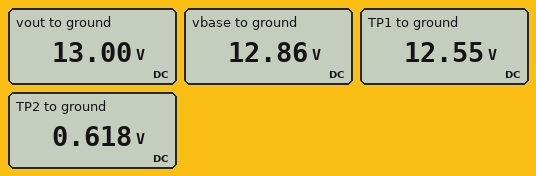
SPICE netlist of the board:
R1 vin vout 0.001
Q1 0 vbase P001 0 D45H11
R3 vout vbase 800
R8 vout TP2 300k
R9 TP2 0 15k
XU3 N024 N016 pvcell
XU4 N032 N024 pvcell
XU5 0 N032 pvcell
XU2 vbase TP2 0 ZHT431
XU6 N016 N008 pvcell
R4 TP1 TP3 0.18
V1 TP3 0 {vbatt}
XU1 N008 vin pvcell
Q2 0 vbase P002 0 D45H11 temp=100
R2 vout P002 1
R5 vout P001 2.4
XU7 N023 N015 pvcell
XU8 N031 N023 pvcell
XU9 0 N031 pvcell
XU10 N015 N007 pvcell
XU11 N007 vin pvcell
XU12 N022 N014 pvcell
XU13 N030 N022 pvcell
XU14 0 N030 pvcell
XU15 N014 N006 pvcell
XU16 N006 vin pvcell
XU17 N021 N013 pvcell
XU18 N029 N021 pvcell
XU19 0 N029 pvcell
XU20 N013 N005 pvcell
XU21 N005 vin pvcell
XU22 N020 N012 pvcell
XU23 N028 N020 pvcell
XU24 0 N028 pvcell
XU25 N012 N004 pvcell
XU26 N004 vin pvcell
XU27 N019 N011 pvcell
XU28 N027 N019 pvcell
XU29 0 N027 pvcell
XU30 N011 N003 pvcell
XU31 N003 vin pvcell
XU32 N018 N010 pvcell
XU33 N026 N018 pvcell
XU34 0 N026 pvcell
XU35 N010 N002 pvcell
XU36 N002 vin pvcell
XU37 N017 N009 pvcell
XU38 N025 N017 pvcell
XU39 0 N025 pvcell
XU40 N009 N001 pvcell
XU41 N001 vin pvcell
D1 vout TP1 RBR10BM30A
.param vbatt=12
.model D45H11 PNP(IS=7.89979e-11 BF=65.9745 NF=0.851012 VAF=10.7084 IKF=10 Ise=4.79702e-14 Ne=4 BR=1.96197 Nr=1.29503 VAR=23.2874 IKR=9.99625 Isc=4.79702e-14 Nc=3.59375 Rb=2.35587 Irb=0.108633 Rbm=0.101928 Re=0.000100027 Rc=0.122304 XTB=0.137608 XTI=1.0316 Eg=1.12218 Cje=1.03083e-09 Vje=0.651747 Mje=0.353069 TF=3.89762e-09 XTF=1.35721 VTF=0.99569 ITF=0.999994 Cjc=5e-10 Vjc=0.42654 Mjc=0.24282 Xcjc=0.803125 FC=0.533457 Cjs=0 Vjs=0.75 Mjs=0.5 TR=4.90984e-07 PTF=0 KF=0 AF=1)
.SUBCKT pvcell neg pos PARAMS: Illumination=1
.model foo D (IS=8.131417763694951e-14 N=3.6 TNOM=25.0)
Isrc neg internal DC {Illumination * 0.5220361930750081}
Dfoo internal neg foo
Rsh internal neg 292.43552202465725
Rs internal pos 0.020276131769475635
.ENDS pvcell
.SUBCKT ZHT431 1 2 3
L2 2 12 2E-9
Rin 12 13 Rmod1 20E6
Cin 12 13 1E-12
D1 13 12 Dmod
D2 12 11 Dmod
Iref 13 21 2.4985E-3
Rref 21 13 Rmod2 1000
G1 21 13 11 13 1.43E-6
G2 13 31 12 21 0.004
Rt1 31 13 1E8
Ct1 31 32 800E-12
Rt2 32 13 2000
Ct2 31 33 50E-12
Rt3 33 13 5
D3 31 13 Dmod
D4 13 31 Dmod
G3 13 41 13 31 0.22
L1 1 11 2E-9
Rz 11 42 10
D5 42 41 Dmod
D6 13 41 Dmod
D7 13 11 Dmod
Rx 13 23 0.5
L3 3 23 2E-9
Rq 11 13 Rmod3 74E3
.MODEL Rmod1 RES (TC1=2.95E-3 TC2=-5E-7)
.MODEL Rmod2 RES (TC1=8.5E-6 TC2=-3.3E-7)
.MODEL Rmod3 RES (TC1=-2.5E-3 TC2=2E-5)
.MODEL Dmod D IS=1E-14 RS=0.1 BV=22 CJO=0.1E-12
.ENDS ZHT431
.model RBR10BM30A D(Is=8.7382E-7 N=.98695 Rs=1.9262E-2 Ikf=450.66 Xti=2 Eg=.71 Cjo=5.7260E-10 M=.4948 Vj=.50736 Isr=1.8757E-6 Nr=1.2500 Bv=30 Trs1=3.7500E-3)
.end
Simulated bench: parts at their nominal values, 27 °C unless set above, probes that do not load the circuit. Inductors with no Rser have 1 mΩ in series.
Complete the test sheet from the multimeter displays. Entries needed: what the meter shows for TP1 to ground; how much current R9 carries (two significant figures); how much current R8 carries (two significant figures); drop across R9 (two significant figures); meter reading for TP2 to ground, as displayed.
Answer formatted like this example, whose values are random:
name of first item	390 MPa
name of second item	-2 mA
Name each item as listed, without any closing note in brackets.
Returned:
what the meter shows for TP1 to ground	12.55 V
how much current R9 carries	41 µA
how much current R8 carries	41 µA
drop across R9	620 mV
meter reading for TP2 to ground, as displayed	0.618 V
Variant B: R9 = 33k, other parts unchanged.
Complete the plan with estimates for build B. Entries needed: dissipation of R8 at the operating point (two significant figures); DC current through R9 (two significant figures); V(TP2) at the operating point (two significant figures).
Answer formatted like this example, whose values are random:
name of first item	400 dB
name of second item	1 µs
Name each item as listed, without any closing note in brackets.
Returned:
dissipation of R8 at the operating point	460 µW
DC current through R9	39 µA
V(TP2) at the operating point	1.3 V
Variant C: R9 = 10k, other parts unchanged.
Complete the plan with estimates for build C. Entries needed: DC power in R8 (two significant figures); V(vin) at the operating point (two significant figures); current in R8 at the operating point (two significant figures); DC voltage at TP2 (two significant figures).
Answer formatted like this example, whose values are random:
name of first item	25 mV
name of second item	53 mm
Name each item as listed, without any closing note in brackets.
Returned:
DC power in R8	530 µW
V(vin) at the operating point	13 V
current in R8 at the operating point	42 µA
DC voltage at TP2	420 mV
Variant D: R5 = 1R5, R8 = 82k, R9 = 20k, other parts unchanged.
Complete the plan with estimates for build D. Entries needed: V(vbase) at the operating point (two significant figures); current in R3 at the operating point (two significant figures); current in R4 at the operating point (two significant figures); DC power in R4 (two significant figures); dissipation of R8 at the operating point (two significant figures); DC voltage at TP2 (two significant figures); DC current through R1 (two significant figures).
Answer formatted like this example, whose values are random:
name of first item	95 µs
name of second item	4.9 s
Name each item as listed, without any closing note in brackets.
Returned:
V(vbase) at the operating point	11 V
current in R3 at the operating point	1.9 mA
current in R4 at the operating point	1.7 A
DC power in R4	530 mW
dissipation of R8 at the operating point	1.3 mW
DC voltage at TP2	2.5 V
DC current through R1	3.5 A
